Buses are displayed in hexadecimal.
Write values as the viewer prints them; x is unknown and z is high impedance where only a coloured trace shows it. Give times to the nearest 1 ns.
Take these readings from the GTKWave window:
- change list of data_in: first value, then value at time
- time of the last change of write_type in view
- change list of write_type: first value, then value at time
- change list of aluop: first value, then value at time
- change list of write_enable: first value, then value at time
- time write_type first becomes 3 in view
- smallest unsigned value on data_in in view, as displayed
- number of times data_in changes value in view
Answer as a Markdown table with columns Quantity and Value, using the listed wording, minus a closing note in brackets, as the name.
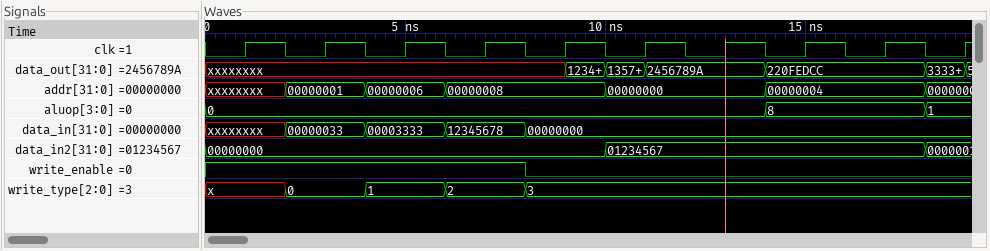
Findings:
| Quantity | Value |
|---|---|
| change list of data_in: first value, then value at time | xxxxxxxx, 00000033 at 2 ns, 00003333 at 4 ns, 12345678 at 6 ns, 00000000 at 8 ns |
| time of the last change of write_type in view | 8 ns |
| change list of write_type: first value, then value at time | x, 0 at 2 ns, 1 at 4 ns, 2 at 6 ns, 3 at 8 ns |
| change list of aluop: first value, then value at time | 0, 8 at 14 ns, 1 at 18 ns |
| change list of write_enable: first value, then value at time | 1, 0 at 8 ns |
| time write_type first becomes 3 in view | 8 ns |
| smallest unsigned value on data_in in view, as displayed | 00000000 |
| number of times data_in changes value in view | 4 |
